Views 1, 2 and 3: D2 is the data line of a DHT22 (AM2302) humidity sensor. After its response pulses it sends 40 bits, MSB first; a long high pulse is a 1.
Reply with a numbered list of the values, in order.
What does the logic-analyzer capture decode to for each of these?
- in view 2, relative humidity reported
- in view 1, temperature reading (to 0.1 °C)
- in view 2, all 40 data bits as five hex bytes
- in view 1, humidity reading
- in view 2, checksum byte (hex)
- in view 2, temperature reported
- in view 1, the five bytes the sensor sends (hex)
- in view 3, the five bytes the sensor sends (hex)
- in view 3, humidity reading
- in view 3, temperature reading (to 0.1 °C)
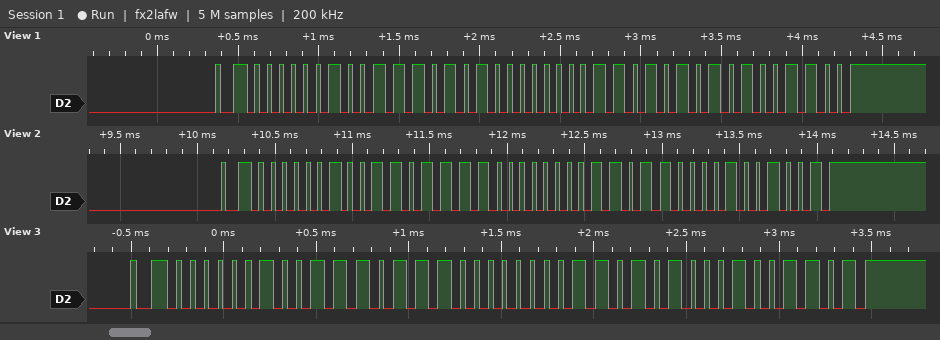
1. 62.3 %
2. 21.3 °C
3. 02 6F 00 D8 49
4. 62.9 %
5. 0x49
6. 21.6 °C
7. 02 75 00 D5 4C
8. 02 77 00 D4 4D
9. 63.1 %
10. 21.2 °C
